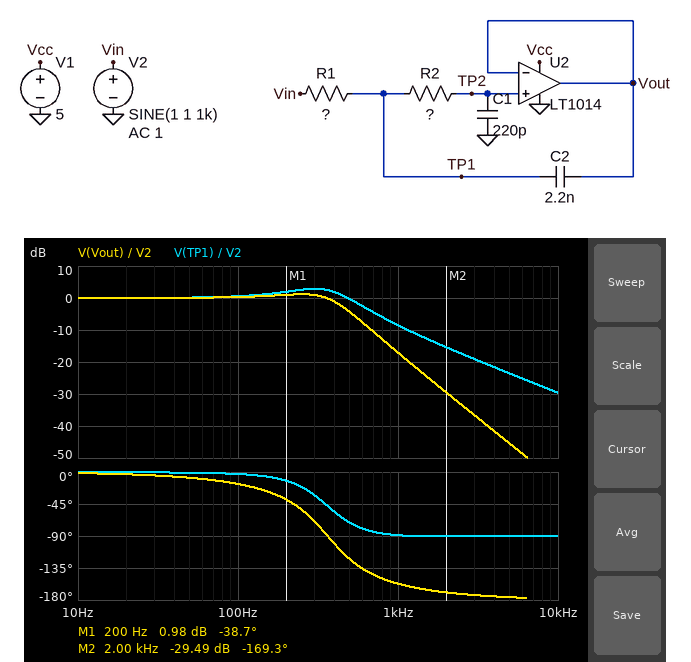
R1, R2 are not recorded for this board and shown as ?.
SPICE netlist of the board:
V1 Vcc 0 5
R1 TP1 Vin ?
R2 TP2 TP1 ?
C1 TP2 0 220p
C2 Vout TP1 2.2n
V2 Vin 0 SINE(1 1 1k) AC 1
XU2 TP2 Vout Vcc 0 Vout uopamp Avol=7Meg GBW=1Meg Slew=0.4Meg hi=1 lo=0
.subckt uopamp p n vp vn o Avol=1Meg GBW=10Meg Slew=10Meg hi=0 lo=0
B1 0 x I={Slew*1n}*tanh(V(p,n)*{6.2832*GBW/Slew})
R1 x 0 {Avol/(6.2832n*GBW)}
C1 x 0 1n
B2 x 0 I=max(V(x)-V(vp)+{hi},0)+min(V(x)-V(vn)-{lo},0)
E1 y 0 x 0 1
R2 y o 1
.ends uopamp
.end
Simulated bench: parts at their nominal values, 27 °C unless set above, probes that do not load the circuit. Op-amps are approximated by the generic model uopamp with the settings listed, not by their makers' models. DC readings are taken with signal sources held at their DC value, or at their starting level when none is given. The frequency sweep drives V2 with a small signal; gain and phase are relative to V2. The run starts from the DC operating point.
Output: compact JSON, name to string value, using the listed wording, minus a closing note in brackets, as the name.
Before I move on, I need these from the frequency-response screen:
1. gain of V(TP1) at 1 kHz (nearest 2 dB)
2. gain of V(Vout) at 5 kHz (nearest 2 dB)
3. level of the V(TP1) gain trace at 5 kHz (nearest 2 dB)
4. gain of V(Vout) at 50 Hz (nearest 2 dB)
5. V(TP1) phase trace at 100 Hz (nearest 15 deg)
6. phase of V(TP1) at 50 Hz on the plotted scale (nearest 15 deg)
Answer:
{"gain of V(TP1) at 1 kHz": "-8 dB", "gain of V(Vout) at 5 kHz": "-46 dB", "level of the V(TP1) gain trace at 5 kHz": "-24 dB", "gain of V(Vout) at 50 Hz": "0 dB", "V(TP1) phase trace at 100 Hz": "0 deg", "phase of V(TP1) at 50 Hz on the plotted scale": "0 deg"}
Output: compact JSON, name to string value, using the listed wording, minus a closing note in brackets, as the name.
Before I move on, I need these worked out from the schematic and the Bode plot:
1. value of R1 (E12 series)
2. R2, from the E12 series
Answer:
{"value of R1": "220 kΩ", "R2, from the E12 series": "1.8 MΩ"}
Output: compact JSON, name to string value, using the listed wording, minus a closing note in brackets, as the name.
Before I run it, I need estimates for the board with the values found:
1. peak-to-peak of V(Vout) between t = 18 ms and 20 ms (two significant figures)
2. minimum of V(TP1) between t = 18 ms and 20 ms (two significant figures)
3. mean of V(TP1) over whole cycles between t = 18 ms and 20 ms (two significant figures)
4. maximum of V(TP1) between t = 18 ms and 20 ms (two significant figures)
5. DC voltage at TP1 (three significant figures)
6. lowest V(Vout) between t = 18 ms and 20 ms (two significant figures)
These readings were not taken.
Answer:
{"peak-to-peak of V(Vout) between t = 18 ms and 20 ms": "280 mV", "minimum of V(TP1) between t = 18 ms and 20 ms": "620 mV", "mean of V(TP1) over whole cycles between t = 18 ms and 20 ms": "1.0 V", "maximum of V(TP1) between t = 18 ms and 20 ms": "1.4 V", "DC voltage at TP1": "1.00 V", "lowest V(Vout) between t = 18 ms and 20 ms": "860 mV"}
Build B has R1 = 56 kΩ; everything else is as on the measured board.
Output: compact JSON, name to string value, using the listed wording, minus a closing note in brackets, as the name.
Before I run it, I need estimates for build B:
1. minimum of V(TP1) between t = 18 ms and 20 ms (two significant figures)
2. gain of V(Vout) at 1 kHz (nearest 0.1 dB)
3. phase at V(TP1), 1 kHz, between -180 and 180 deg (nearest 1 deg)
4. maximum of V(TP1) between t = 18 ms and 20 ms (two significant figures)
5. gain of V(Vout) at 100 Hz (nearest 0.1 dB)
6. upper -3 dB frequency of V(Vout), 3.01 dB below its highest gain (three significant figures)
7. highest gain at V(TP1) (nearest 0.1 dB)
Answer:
{"minimum of V(TP1) between t = 18 ms and 20 ms": "17 mV", "gain of V(Vout) at 1 kHz": "-8.7 dB", "phase at V(TP1), 1 kHz, between -180 and 180 deg": "-42 deg", "maximum of V(TP1) between t = 18 ms and 20 ms": "2.0 V", "gain of V(Vout) at 100 Hz": "-0.1 dB", "upper -3 dB frequency of V(Vout), 3.01 dB below its highest gain": "518 Hz", "highest gain at V(TP1)": "1.2 dB"}
